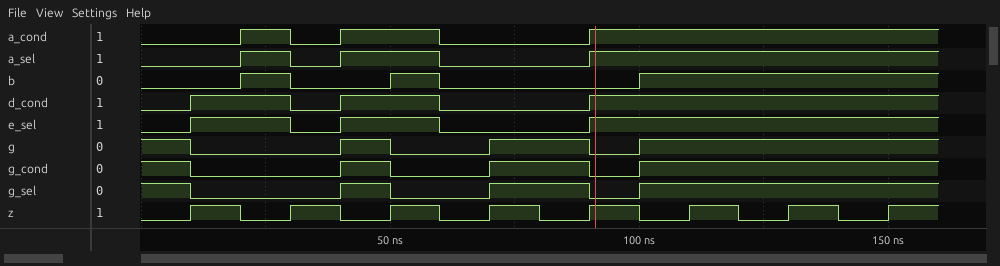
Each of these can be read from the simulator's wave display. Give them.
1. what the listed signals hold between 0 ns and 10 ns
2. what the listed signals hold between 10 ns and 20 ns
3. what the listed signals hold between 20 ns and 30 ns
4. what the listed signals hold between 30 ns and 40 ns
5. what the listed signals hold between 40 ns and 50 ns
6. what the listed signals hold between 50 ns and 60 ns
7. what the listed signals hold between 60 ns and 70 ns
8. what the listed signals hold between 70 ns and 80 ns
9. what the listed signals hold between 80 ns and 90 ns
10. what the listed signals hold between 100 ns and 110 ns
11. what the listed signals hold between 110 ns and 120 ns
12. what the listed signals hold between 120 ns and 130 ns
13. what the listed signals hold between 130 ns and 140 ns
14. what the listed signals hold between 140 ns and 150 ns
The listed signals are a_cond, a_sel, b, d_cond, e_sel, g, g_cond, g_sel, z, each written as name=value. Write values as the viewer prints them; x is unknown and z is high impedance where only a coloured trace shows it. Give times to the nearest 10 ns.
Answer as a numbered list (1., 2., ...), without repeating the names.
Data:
1. a_cond=0, a_sel=0, b=0, d_cond=0, e_sel=0, g=1, g_cond=1, g_sel=1, z=0
2. a_cond=0, a_sel=0, b=0, d_cond=1, e_sel=1, g=0, g_cond=0, g_sel=0, z=1
3. a_cond=1, a_sel=1, b=1, d_cond=1, e_sel=1, g=0, g_cond=0, g_sel=0, z=0
4. a_cond=0, a_sel=0, b=0, d_cond=0, e_sel=0, g=0, g_cond=0, g_sel=0, z=1
5. a_cond=1, a_sel=1, b=0, d_cond=1, e_sel=1, g=1, g_cond=1, g_sel=1, z=0
6. a_cond=1, a_sel=1, b=1, d_cond=1, e_sel=1, g=0, g_cond=0, g_sel=0, z=1
7. a_cond=0, a_sel=0, b=0, d_cond=0, e_sel=0, g=0, g_cond=0, g_sel=0, z=0
8. a_cond=0, a_sel=0, b=0, d_cond=0, e_sel=0, g=1, g_cond=1, g_sel=1, z=1
9. a_cond=0, a_sel=0, b=0, d_cond=0, e_sel=0, g=1, g_cond=1, g_sel=1, z=0
10. a_cond=1, a_sel=1, b=1, d_cond=1, e_sel=1, g=1, g_cond=1, g_sel=1, z=0
11. a_cond=1, a_sel=1, b=1, d_cond=1, e_sel=1, g=1, g_cond=1, g_sel=1, z=1
12. a_cond=1, a_sel=1, b=1, d_cond=1, e_sel=1, g=1, g_cond=1, g_sel=1, z=0
13. a_cond=1, a_sel=1, b=1, d_cond=1, e_sel=1, g=1, g_cond=1, g_sel=1, z=1
14. a_cond=1, a_sel=1, b=1, d_cond=1, e_sel=1, g=1, g_cond=1, g_sel=1, z=0
